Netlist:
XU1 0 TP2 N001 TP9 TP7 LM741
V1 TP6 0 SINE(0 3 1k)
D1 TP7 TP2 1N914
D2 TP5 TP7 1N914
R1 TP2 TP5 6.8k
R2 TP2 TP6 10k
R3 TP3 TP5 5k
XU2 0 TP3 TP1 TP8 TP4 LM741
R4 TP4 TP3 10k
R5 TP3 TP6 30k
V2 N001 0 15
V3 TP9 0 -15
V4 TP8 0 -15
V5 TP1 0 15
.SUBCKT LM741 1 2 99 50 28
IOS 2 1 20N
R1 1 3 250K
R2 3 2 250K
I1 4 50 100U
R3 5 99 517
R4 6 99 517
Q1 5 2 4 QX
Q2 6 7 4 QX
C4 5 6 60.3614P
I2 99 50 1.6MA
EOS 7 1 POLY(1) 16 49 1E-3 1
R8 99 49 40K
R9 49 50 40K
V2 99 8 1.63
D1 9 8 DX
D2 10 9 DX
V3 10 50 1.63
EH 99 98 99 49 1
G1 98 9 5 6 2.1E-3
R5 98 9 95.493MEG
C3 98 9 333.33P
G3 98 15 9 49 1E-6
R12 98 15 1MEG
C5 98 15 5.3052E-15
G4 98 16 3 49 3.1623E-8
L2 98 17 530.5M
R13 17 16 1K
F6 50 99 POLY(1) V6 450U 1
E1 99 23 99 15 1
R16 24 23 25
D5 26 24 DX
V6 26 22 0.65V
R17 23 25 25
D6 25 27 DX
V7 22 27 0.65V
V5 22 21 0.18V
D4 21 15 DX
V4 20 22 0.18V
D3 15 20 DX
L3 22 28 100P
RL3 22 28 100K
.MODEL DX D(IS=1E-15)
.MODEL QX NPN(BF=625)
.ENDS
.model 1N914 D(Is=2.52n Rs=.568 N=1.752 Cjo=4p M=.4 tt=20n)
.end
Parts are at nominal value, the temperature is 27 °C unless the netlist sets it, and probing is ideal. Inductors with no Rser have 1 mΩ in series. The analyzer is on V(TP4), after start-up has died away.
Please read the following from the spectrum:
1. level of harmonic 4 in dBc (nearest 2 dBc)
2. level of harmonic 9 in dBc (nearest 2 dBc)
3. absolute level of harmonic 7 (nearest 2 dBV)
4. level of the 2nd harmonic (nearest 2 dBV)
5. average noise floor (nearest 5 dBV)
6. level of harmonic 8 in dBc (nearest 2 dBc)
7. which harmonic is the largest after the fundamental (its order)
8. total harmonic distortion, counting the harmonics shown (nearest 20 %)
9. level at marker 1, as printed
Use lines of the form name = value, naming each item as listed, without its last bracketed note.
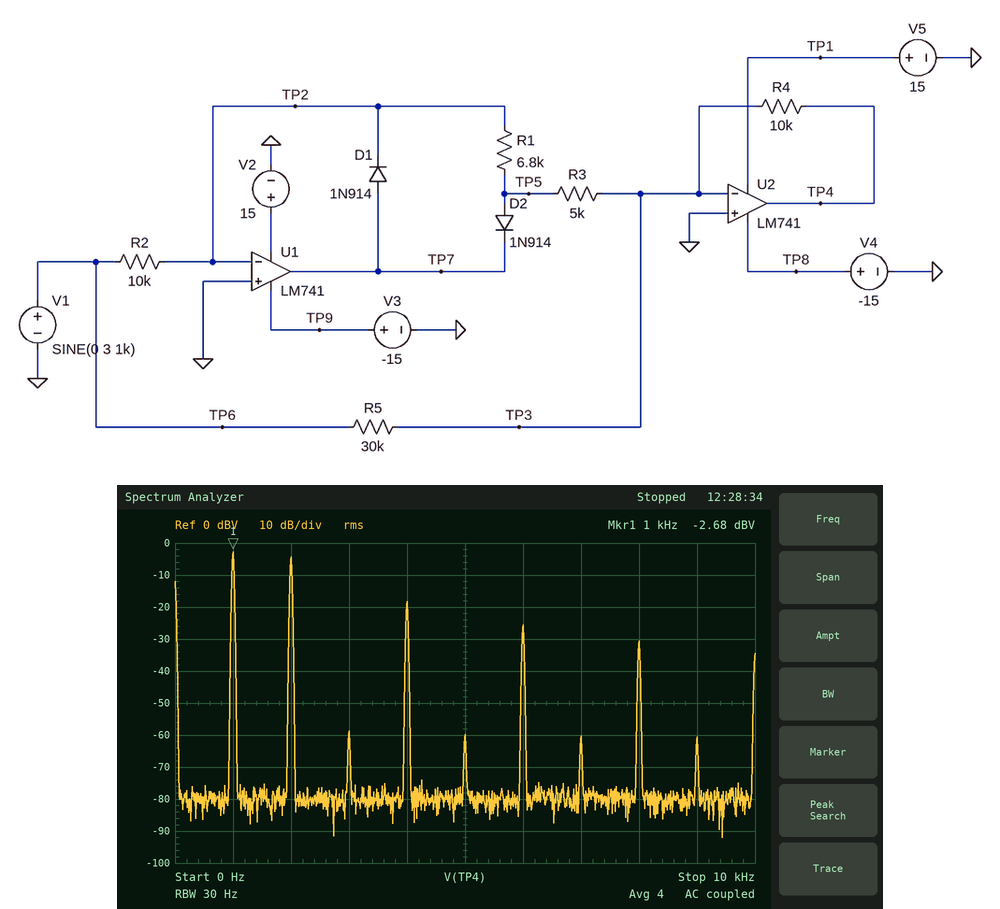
level of harmonic 4 in dBc = -16 dBc
level of harmonic 9 in dBc = -58 dBc
absolute level of harmonic 7 = -60 dBV
level of the 2nd harmonic = -4 dBV
average noise floor = -80 dBV
level of harmonic 8 in dBc = -28 dBc
which harmonic is the largest after the fundamental = 2
total harmonic distortion, counting the harmonics shown = 80 %
level at marker 1, as printed = -2.68 dBV
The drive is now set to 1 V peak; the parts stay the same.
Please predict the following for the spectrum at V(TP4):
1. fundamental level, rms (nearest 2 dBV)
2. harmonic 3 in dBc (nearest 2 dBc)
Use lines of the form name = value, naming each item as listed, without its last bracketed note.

fundamental level, rms = -12 dBV
harmonic 3 in dBc = -48 dBc
